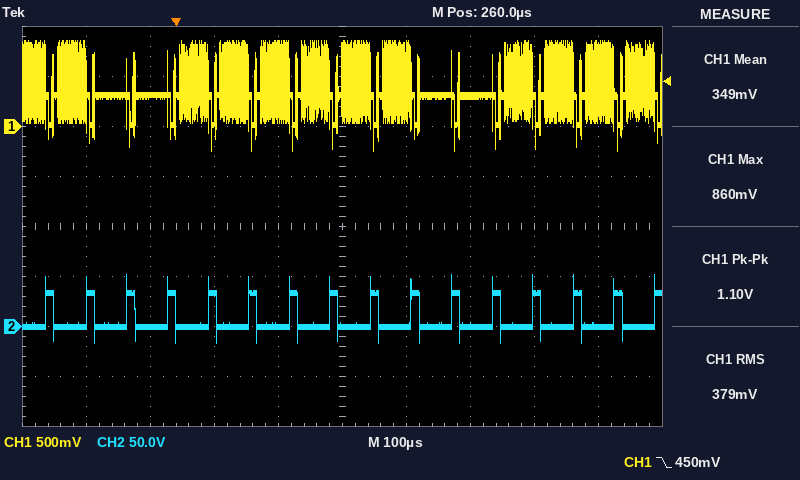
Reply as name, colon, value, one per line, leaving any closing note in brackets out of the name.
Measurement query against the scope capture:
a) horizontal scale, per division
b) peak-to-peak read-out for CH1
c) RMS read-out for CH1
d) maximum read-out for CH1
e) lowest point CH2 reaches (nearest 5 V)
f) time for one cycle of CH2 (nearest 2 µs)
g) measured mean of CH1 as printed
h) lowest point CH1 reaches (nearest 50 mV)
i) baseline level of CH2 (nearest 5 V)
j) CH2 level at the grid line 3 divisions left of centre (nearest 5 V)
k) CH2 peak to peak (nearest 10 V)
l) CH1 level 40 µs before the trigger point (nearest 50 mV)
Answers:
horizontal scale, per division: 100 µs
peak-to-peak read-out for CH1: 1.10 V
RMS read-out for CH1: 379 mV
maximum read-out for CH1: 860 mV
lowest point CH2 reaches: -15 V
time for one cycle of CH2: 64 µs
measured mean of CH1 as printed: 349 mV
lowest point CH1 reaches: -250 mV
baseline level of CH2: 0 V
CH2 level at the grid line 3 divisions left of centre: 0 V
CH2 peak to peak: 70 V
CH1 level 40 µs before the trigger point: 300 mV
